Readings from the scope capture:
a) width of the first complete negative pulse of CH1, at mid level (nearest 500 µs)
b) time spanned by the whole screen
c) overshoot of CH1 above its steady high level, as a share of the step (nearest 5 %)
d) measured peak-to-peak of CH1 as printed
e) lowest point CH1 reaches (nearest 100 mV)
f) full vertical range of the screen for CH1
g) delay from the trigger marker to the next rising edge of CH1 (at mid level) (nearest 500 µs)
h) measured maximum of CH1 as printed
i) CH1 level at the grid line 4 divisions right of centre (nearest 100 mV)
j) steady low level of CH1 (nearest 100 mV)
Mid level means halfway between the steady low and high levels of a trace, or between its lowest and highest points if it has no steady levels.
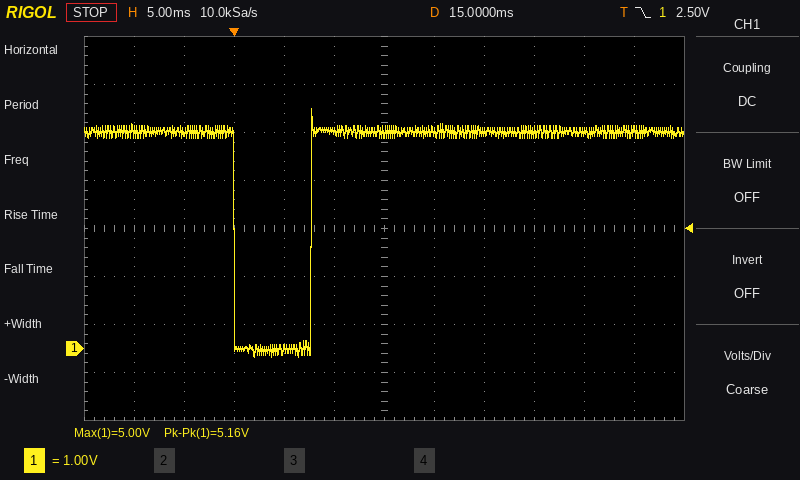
7.5 ms
60 ms
10 %
5.16 V
-200 mV
8 V
7.5 ms
5.00 V
4.5 V
0.0 V
